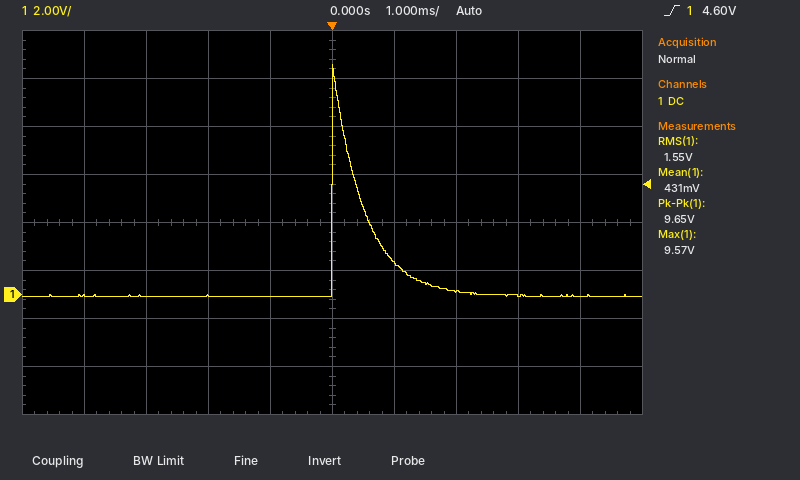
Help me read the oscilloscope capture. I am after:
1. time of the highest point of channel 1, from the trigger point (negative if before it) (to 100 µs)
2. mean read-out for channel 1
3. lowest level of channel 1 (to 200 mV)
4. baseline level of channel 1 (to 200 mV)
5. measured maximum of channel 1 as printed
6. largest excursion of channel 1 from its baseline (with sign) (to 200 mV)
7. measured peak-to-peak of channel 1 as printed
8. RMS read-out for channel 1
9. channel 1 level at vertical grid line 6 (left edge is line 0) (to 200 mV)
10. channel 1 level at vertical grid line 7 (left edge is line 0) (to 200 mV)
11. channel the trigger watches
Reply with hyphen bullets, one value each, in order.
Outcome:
- 0.0 ms
- 431 mV
- 0.0 V
- 0.0 V
- 9.57 V
- +9.6 V
- 9.65 V
- 1.55 V
- 1.4 V
- 200 mV
- channel 1
